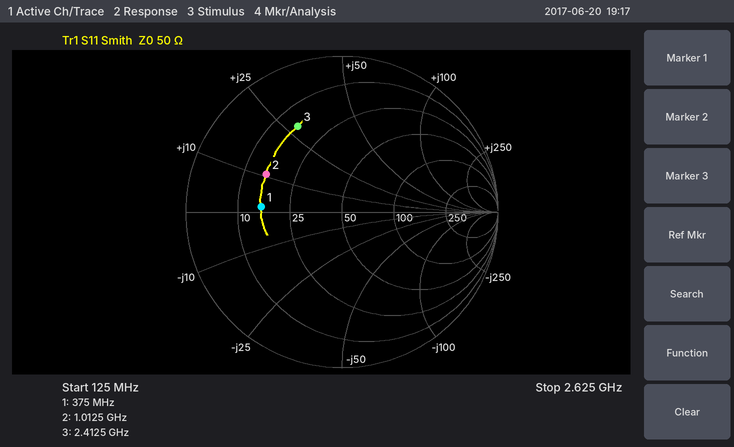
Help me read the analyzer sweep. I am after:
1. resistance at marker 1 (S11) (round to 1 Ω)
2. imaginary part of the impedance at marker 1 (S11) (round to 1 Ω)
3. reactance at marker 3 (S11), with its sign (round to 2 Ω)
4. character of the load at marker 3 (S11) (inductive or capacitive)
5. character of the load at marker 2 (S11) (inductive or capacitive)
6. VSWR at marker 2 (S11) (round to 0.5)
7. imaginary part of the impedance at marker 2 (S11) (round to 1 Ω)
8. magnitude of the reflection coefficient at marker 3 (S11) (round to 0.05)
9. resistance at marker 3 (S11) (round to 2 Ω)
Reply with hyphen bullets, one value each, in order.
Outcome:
- 16 Ω
- +1 Ω
- +28 Ω
- inductive
- inductive
- 3.5
- +11 Ω
- 0.60
- 16 Ω
